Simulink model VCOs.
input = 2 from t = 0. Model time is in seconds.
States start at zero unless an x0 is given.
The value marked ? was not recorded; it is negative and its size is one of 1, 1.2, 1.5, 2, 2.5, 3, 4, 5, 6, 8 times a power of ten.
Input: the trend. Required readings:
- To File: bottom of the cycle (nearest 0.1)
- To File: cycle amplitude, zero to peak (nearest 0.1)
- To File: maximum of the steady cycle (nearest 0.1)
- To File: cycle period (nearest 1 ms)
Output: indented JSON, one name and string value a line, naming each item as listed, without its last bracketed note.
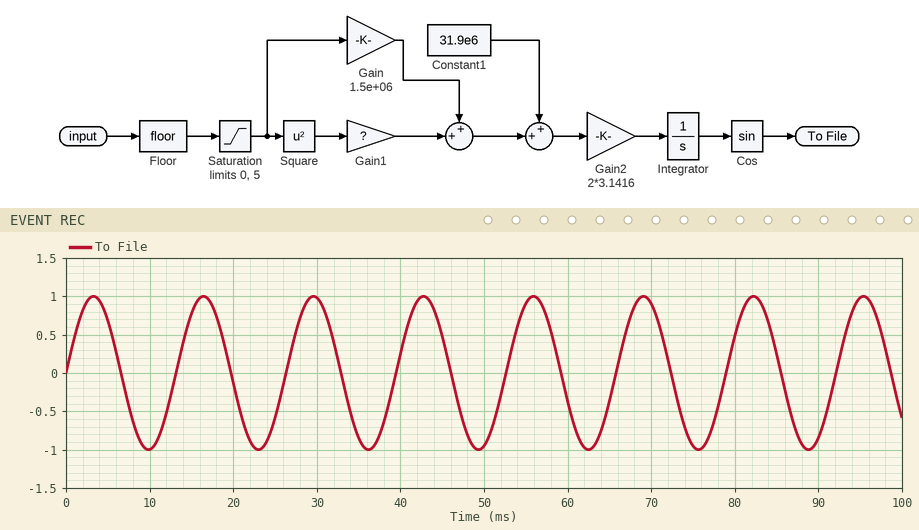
{
  "To File: bottom of the cycle": "-1.0",
  "To File: cycle amplitude, zero to peak": "1.0",
  "To File: maximum of the steady cycle": "1.0",
  "To File: cycle period": "13 ms"
}
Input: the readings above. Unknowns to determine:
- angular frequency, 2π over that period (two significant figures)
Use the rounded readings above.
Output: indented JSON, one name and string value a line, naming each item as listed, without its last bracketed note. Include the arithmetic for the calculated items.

{
  "angular frequency, 2π over that period": "2π / 13 = 0.48 rad/ms"
}
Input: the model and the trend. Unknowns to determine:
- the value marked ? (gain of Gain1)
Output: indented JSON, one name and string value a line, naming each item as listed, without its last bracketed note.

{
  "the value marked ?": "-600000"
}
